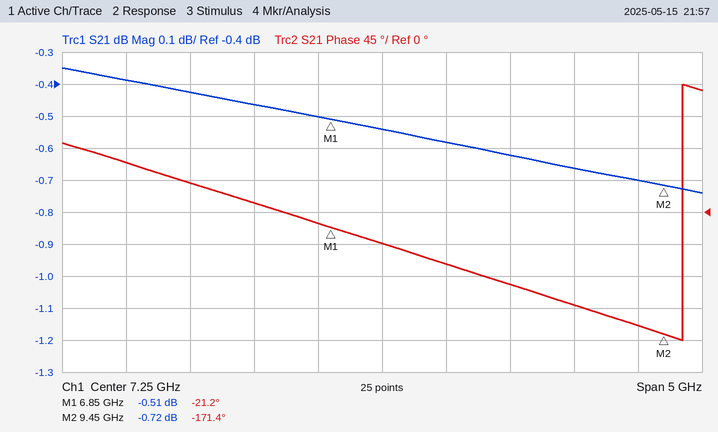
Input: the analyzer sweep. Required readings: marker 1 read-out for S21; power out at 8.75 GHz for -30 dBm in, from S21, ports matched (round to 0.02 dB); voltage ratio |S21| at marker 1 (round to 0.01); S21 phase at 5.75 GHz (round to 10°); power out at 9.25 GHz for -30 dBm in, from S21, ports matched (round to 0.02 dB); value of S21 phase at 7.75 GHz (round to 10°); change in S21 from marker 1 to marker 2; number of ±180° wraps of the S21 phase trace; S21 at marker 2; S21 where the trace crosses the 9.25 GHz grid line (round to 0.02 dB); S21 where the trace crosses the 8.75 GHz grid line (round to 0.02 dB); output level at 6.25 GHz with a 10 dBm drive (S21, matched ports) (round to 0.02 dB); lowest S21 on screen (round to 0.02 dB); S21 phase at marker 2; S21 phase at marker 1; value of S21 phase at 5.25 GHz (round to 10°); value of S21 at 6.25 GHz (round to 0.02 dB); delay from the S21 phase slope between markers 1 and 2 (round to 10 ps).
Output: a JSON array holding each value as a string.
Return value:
["-0.51 dB", "-30.66 dBm", "0.94", "40°", "-30.70 dBm", "-70°", "-0.21 dB", "1", "-0.72 dB", "-0.70 dB", "-0.66 dB", "9.54 dBm", "-0.74 dB", "-171.4°", "-21.2°", "70°", "-0.46 dB", "160 ps"]
